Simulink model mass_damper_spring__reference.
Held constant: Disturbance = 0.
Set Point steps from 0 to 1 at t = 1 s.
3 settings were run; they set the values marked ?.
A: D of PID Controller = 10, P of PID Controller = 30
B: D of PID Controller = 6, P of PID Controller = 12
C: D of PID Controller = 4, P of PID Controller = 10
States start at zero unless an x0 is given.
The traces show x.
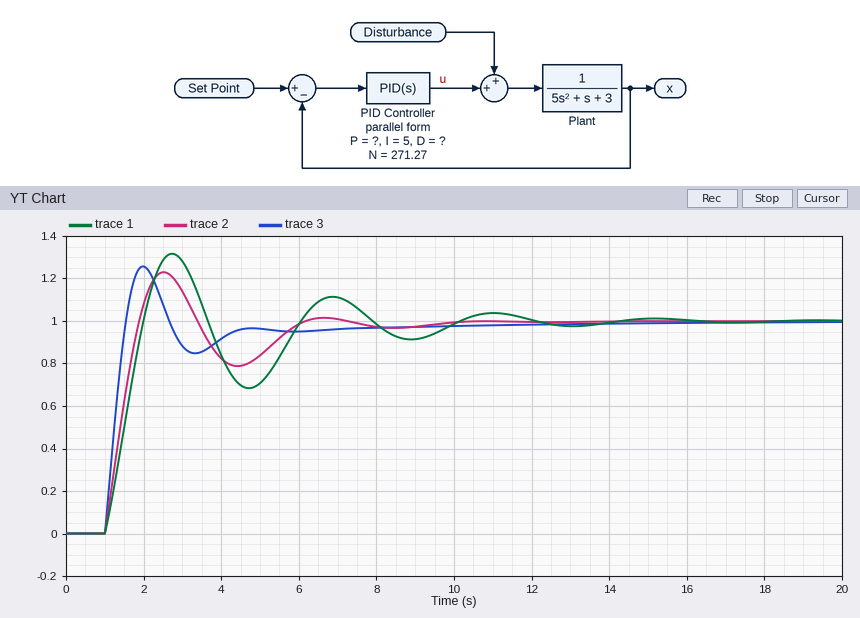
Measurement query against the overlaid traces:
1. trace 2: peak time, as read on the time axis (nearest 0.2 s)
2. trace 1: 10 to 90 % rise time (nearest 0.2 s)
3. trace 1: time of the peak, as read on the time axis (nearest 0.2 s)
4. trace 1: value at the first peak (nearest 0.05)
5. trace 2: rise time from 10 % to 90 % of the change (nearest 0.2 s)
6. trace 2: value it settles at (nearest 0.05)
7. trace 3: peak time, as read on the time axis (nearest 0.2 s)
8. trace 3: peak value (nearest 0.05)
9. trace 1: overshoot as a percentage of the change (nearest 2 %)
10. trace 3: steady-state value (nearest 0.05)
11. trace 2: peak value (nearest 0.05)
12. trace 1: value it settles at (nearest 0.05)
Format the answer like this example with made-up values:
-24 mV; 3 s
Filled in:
2.6 s; 0.8 s; 2.8 s; 1.30; 0.6 s; 1.00; 2.0 s; 1.25; 32 %; 1.00; 1.25; 1.00
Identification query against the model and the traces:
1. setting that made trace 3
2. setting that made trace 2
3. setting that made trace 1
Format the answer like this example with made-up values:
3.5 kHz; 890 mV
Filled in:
A; B; C
